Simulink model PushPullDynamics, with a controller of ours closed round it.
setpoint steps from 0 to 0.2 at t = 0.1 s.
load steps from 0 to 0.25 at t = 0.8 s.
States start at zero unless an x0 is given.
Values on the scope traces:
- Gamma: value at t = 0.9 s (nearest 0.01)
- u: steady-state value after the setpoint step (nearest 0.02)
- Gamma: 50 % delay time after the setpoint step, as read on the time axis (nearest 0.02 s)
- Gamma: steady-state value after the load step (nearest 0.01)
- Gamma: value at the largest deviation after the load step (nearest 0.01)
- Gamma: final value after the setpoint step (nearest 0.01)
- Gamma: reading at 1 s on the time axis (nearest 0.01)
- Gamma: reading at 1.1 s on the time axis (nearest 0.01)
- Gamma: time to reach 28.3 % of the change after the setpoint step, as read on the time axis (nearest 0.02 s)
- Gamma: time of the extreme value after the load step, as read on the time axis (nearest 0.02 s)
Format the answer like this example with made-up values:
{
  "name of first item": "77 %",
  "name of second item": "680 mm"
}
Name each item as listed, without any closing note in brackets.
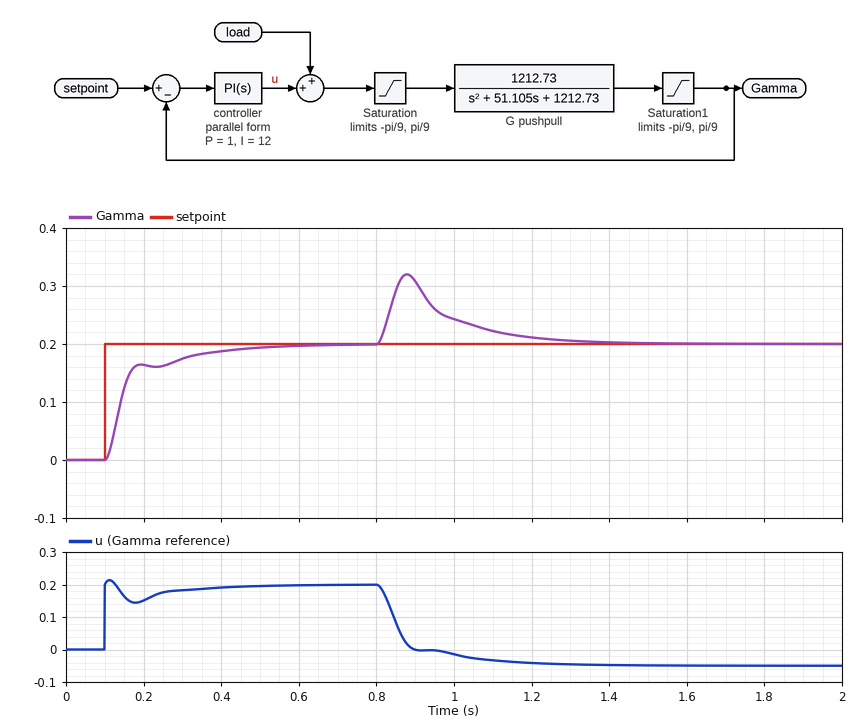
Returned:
{
  "Gamma: value at t = 0.9 s": "0.31",
  "u: steady-state value after the setpoint step": "0.20",
  "Gamma: 50 % delay time after the setpoint step, as read on the time axis": "0.14 s",
  "Gamma: steady-state value after the load step": "0.20",
  "Gamma: value at the largest deviation after the load step": "0.32",
  "Gamma: final value after the setpoint step": "0.20",
  "Gamma: reading at 1 s on the time axis": "0.24",
  "Gamma: reading at 1.1 s on the time axis": "0.22",
  "Gamma: time to reach 28.3 % of the change after the setpoint step, as read on the time axis": "0.12 s",
  "Gamma: time of the extreme value after the load step, as read on the time axis": "0.88 s"
}
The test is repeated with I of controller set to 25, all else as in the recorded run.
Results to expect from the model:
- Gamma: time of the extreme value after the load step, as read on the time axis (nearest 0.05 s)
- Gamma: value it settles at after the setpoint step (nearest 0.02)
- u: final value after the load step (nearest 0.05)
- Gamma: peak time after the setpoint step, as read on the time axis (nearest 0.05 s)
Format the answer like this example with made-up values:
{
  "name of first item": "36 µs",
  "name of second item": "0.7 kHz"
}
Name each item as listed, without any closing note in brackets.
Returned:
{
  "Gamma: time of the extreme value after the load step, as read on the time axis": "0.85 s",
  "Gamma: value it settles at after the setpoint step": "0.20",
  "u: final value after the load step": "-0.05",
  "Gamma: peak time after the setpoint step, as read on the time axis": "0.20 s"
}
